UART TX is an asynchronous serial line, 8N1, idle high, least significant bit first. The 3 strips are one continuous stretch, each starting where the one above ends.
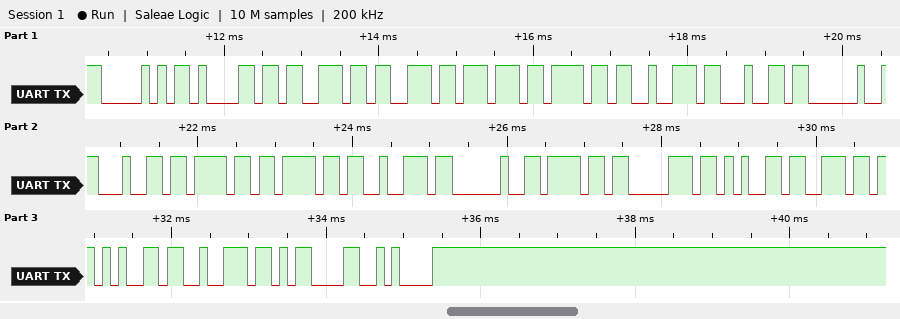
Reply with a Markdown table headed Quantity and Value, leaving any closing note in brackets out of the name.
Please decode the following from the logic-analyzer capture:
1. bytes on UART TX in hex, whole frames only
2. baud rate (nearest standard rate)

| Quantity | Value |
|---|---|
| bytes on UART TX in hex, whole frames only | 50 61 73 73 77 6F 72 64 20 64 6F 6F 72 20 6F 70 65 6E 65 72 0D 0A |
| baud rate | 9600 baud |
